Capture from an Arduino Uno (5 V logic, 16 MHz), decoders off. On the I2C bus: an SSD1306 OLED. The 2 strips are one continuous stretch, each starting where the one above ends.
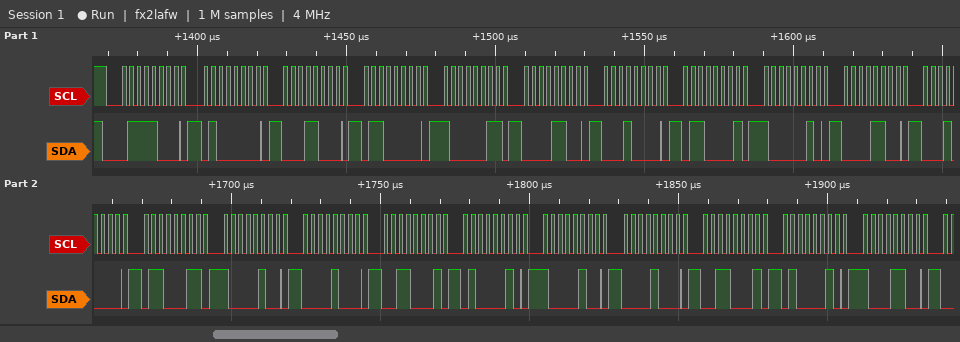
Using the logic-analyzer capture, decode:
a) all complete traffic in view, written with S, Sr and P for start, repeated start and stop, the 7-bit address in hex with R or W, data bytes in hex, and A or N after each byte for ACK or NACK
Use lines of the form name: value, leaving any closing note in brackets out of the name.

all complete traffic in view, written with S, Sr and P for start, repeated start and stop, the 7-bit address in hex with R or W, data bytes in hex, and A or N after each byte for ACK or NACK: S 3CW A 40 A 18 A 60 A 83 A 0C A 10 A 61 A 82 A 0C A 10 A 63 A 84 A 08 A 31 A 42 A 84 A 08 A 31 A 42 A 8C A
